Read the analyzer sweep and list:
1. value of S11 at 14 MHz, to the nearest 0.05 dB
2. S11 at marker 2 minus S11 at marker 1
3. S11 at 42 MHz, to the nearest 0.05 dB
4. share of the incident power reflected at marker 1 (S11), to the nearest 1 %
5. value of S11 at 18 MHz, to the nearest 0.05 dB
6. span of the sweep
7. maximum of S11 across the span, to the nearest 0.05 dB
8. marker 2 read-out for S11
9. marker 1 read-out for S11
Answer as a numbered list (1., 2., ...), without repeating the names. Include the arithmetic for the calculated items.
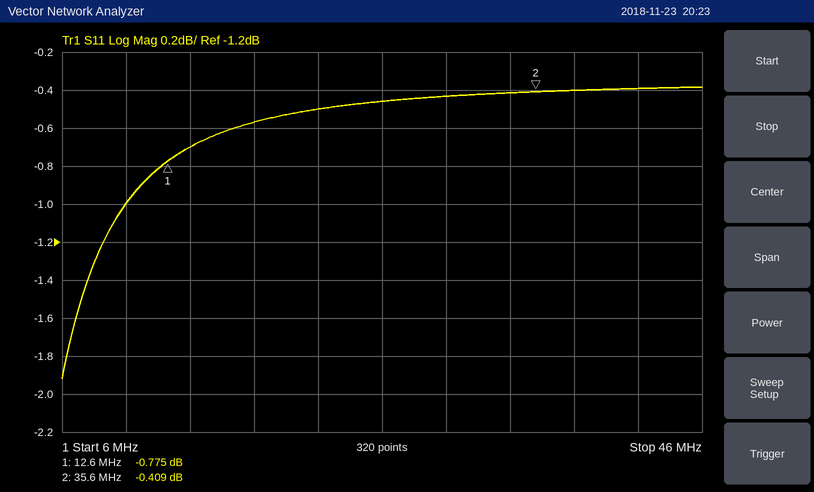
1. -0.70 dB
2. -0.409 − (-0.775) = 0.366 dB
3. -0.40 dB
4. 10^(-0.775/10) ≈ 84 %
5. -0.55 dB
6. 40 MHz
7. -0.40 dB
8. -0.409 dB
9. -0.775 dB
